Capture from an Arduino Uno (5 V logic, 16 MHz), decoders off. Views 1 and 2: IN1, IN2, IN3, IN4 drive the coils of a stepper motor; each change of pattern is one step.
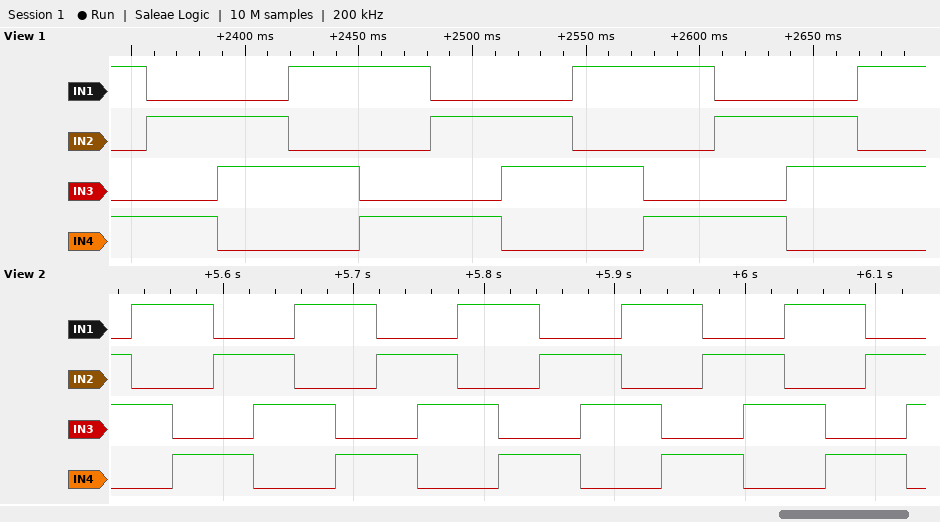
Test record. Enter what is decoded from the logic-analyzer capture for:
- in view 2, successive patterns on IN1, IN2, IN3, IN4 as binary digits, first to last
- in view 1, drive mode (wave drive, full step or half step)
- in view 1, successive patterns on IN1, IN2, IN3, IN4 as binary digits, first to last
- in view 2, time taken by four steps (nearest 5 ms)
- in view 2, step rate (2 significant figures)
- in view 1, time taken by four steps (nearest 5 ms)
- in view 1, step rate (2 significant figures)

0110 1010 1001 0101 0110 1010 1001 0101 0110 1010 1001 0101 0110 1010 1001 0101 0110 1010 1001 0101 0110
full step
1001 0101 0110 1010 1001 0101 0110 1010 1001 0101 0110 1010
125 ms
32 steps/s
125 ms
32 steps/s
